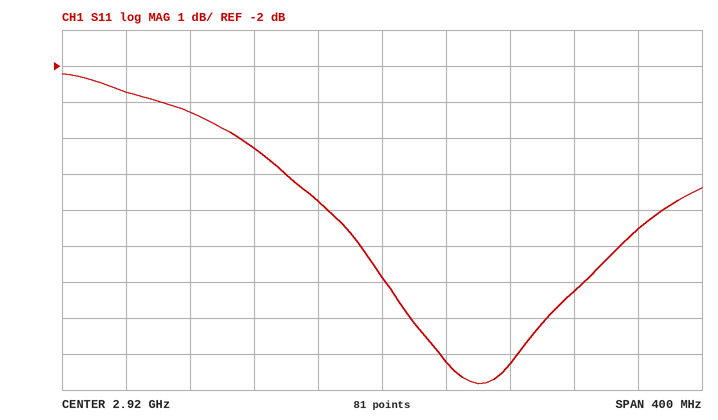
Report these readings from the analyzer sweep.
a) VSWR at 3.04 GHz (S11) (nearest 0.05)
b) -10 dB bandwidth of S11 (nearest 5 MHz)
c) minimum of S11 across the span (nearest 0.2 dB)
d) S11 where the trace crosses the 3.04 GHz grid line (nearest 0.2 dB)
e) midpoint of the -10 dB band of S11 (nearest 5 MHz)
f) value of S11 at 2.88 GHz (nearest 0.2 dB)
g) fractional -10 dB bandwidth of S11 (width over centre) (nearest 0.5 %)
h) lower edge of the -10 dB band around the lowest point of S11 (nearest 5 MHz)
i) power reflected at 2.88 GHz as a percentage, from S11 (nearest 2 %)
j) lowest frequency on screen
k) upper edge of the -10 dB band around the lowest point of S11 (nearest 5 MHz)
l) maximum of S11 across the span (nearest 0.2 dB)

2.25
50 MHz
-10.8 dB
-8.2 dB
2.980 GHz
-5.8 dB
1.5 %
2.955 GHz
26 %
2.72 GHz
3.005 GHz
-2.2 dB
